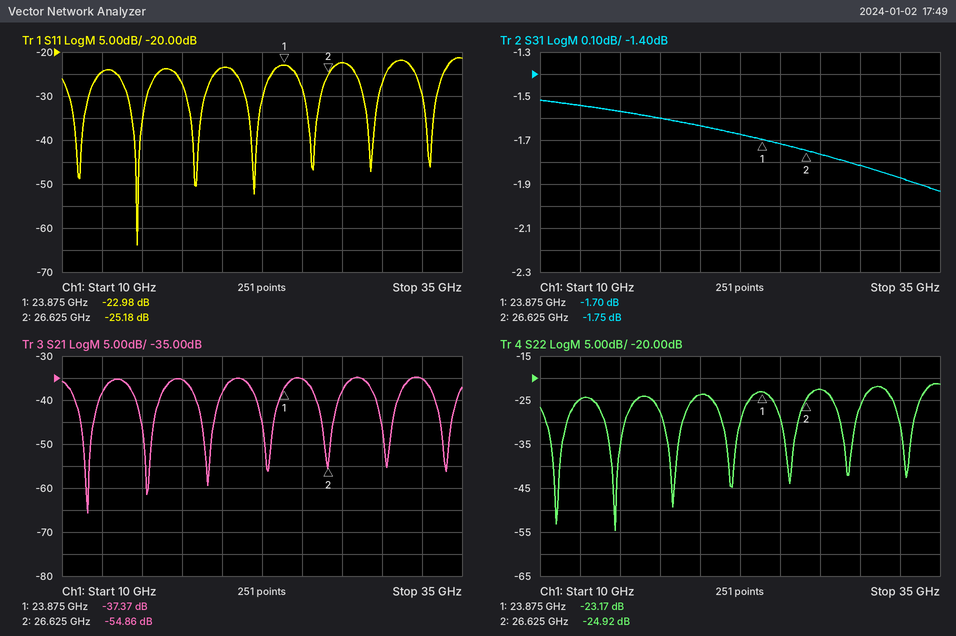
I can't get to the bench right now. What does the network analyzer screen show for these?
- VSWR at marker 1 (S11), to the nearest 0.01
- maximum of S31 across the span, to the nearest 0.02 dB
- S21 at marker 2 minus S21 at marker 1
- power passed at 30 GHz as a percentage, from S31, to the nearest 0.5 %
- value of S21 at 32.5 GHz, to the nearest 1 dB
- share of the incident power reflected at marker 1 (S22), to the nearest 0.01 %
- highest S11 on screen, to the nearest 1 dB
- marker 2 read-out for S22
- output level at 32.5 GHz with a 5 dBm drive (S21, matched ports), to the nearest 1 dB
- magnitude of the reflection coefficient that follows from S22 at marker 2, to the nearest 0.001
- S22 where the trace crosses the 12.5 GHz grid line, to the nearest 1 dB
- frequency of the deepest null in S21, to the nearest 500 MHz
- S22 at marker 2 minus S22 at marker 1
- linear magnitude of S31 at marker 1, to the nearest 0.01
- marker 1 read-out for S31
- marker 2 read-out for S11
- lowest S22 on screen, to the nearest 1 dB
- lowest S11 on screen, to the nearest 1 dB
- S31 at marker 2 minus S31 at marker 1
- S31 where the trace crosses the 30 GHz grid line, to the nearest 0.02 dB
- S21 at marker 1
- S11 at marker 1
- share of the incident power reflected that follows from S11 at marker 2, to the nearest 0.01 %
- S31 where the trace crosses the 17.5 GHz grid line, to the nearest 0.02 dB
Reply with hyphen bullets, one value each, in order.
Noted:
- 1.15
- -1.52 dB
- -17.49 dB
- 66.0 %
- -35 dB
- 0.48 %
- -21 dB
- -24.92 dB
- -30 dBm
- 0.057
- -25 dB
- 11.5 GHz
- -1.75 dB
- 0.82
- -1.70 dB
- -25.18 dB
- -55 dB
- -64 dB
- -0.05 dB
- -1.82 dB
- -37.37 dB
- -22.98 dB
- 0.30 %
- -1.60 dB
